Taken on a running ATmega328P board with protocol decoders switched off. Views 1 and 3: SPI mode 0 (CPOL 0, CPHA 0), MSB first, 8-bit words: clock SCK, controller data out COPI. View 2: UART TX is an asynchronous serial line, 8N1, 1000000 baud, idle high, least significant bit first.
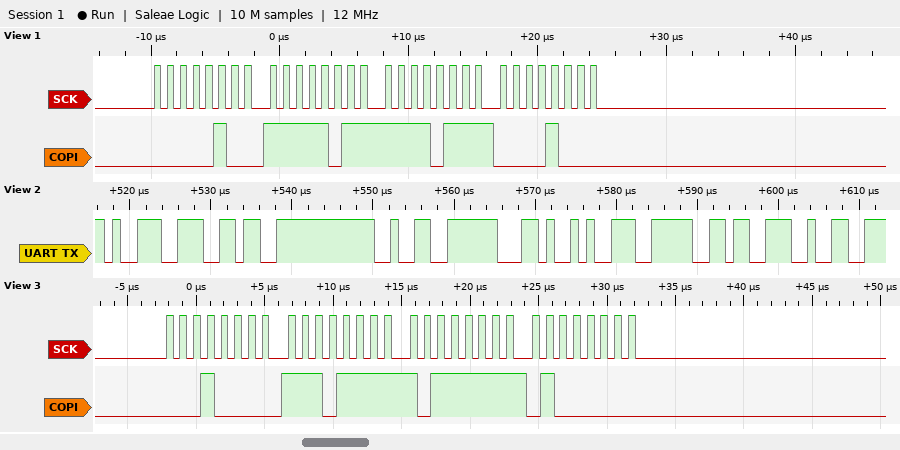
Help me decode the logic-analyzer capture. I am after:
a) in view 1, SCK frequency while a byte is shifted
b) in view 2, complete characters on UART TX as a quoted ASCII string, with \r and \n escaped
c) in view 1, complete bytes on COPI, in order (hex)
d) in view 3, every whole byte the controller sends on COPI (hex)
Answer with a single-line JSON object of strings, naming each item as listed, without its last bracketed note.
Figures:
{"in view 1, SCK frequency while a byte is shifted": "1 MHz", "in view 2, complete characters on UART TX as a quoted ASCII string, with \\r and \\n escaped": "\"962,962\"", "in view 1, complete bytes on COPI, in order": "04 FB F7 08", "in view 3, every whole byte the controller sends on COPI": "10 EF BF 40"}
